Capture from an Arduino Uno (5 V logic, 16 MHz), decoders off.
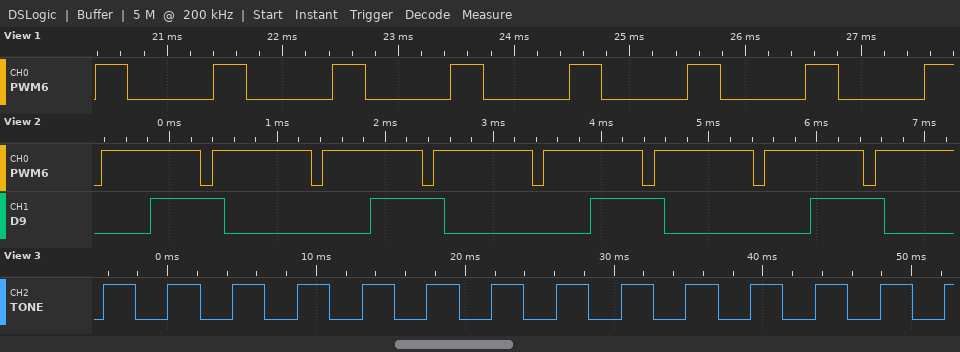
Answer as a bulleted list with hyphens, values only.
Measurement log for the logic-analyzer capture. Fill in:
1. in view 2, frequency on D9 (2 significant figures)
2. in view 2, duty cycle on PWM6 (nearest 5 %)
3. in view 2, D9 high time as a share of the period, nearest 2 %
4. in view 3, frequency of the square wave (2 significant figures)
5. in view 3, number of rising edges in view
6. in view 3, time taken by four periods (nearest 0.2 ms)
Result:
- 490 Hz
- 90 %
- 34 %
- 230 Hz
- 14
- 17.4 ms
